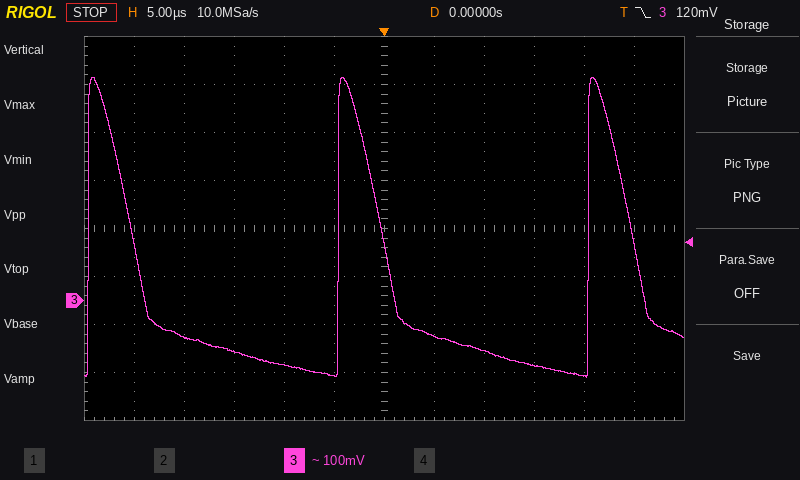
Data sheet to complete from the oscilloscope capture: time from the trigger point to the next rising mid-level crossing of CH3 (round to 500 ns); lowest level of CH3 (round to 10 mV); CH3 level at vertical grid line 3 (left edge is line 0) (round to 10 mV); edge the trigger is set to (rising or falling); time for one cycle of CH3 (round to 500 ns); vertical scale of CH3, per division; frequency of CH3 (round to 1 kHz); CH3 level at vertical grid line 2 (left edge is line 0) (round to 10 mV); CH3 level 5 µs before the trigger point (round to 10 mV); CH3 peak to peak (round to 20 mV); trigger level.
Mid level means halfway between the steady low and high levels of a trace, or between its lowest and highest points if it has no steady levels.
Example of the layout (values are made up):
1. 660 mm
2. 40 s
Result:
1. 20.5 µs
2. -160 mV
3. -110 mV
4. falling
5. 25.0 µs
6. 100 mV
7. 40 kHz
8. -80 mV
9. -160 mV
10. 620 mV
11. 120 mV
